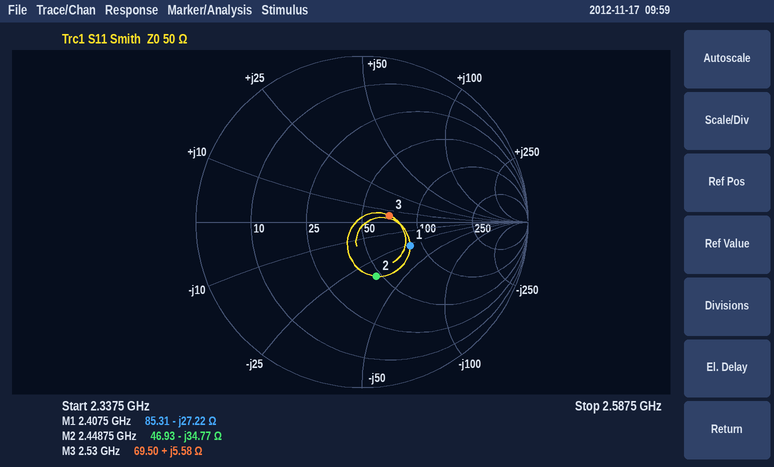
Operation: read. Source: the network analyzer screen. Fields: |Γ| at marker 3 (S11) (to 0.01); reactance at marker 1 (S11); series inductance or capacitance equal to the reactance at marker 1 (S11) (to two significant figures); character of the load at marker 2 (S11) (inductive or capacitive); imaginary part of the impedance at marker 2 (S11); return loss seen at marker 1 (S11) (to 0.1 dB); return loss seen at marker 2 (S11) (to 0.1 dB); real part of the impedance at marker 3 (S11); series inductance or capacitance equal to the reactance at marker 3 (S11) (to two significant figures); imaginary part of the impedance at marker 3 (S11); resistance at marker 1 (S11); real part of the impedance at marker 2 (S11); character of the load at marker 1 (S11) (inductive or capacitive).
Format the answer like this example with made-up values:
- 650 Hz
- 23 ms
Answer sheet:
- 0.17
- -27.22 Ω
- 2.4 pF
- capacitive
- -34.77 Ω
- 9.8 dB
- 9.4 dB
- 69.50 Ω
- 350 pH
- +5.58 Ω
- 85.31 Ω
- 46.93 Ω
- capacitive
